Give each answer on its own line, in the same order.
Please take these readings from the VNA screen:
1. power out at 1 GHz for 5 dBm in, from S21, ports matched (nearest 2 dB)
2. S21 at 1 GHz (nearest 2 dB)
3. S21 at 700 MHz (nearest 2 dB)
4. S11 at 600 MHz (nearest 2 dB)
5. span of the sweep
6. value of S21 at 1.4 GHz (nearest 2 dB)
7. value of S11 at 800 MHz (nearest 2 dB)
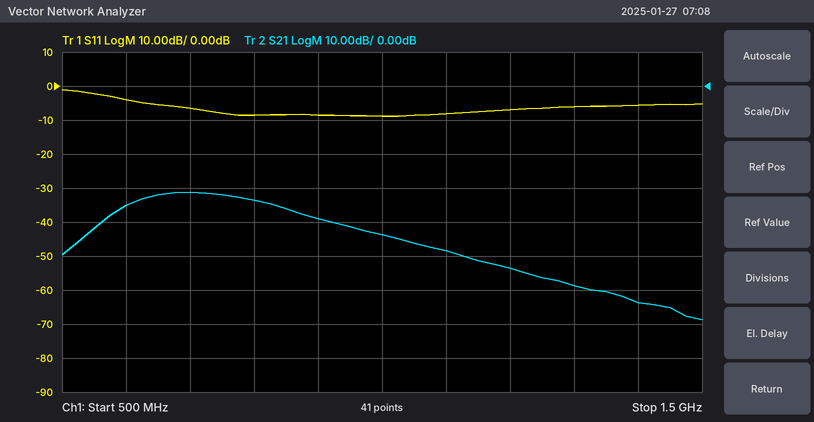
-38 dBm
-44 dB
-32 dB
-4 dB
1 GHz
-64 dB
-8 dB
